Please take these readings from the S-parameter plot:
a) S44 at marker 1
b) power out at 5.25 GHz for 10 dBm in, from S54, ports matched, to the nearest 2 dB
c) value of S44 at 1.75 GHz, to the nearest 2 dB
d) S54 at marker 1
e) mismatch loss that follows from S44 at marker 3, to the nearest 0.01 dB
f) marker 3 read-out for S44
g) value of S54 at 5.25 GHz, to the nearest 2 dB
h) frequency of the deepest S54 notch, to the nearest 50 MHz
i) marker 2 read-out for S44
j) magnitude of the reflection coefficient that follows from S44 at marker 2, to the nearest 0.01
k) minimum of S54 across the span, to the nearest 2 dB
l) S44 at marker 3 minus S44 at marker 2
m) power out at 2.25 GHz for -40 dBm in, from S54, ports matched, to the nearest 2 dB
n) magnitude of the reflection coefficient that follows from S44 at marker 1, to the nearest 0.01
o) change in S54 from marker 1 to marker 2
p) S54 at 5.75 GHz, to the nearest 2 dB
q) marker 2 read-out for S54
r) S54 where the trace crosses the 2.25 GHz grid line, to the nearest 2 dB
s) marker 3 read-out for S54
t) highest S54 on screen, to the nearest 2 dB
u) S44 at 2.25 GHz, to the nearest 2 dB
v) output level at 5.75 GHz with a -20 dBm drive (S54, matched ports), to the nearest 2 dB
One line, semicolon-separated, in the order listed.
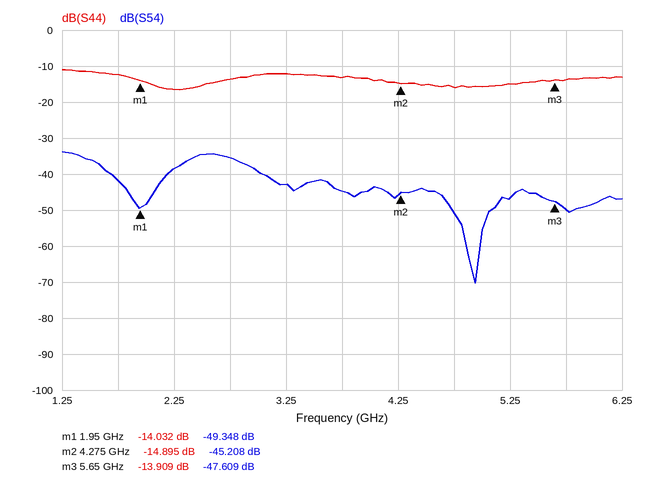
-14.032 dB; -36 dBm; -12 dB; -49.348 dB; 0.18 dB; -13.909 dB; -46 dB; 4.95 GHz; -14.895 dB; 0.18; -70 dB; 0.986 dB; -78 dBm; 0.20; 4.140 dB; -50 dB; -45.208 dB; -38 dB; -47.609 dB; -34 dB; -16 dB; -70 dBm
